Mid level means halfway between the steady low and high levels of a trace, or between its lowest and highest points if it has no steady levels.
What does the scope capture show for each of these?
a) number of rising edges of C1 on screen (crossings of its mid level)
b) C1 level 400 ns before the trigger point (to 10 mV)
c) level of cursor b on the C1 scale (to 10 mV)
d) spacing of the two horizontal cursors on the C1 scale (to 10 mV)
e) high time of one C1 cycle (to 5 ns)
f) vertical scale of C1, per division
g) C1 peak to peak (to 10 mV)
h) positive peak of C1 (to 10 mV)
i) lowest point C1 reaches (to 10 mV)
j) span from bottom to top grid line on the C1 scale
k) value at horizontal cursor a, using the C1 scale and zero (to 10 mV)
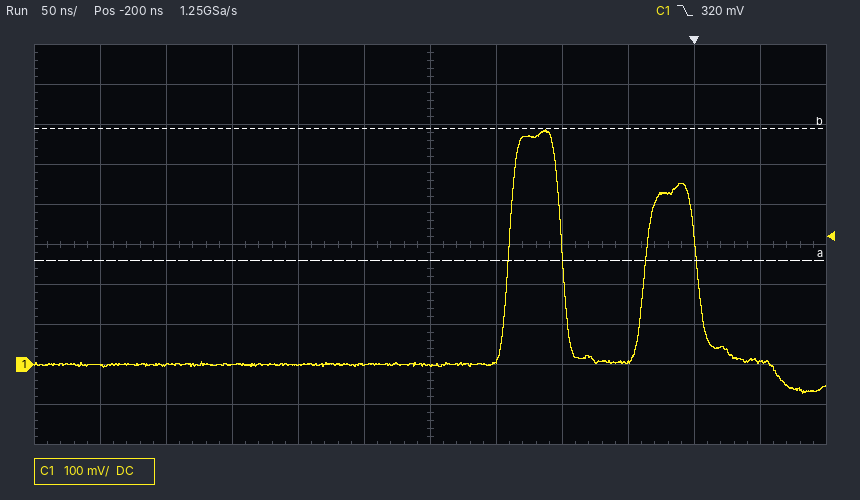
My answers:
2
0 mV
590 mV
330 mV
40 ns
100 mV
660 mV
590 mV
-70 mV
1 V
260 mV
